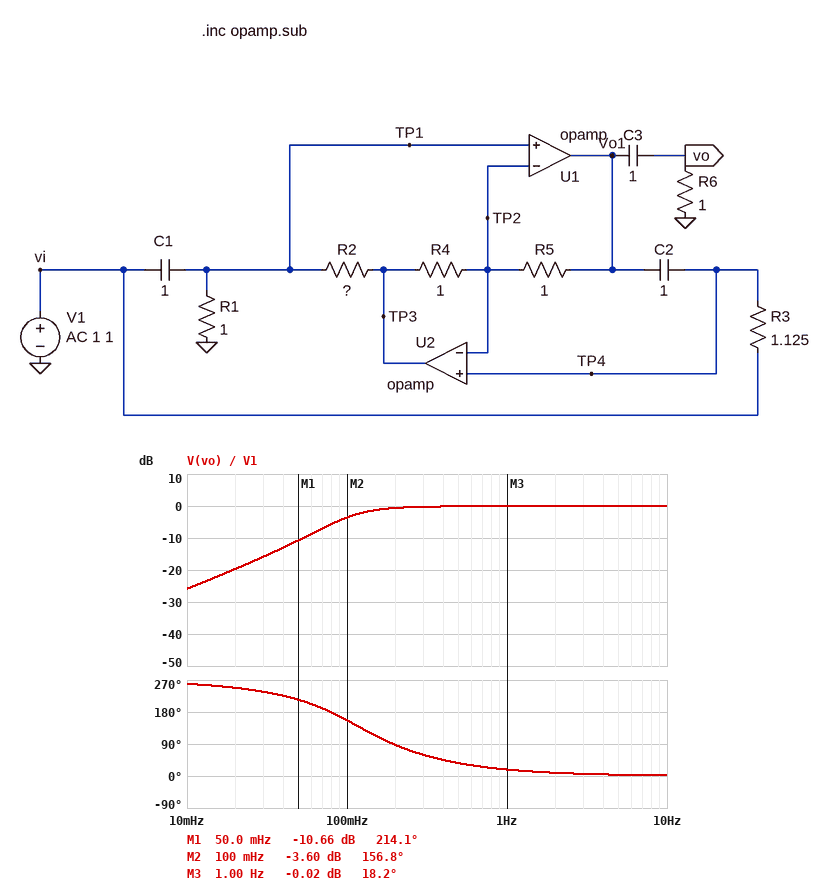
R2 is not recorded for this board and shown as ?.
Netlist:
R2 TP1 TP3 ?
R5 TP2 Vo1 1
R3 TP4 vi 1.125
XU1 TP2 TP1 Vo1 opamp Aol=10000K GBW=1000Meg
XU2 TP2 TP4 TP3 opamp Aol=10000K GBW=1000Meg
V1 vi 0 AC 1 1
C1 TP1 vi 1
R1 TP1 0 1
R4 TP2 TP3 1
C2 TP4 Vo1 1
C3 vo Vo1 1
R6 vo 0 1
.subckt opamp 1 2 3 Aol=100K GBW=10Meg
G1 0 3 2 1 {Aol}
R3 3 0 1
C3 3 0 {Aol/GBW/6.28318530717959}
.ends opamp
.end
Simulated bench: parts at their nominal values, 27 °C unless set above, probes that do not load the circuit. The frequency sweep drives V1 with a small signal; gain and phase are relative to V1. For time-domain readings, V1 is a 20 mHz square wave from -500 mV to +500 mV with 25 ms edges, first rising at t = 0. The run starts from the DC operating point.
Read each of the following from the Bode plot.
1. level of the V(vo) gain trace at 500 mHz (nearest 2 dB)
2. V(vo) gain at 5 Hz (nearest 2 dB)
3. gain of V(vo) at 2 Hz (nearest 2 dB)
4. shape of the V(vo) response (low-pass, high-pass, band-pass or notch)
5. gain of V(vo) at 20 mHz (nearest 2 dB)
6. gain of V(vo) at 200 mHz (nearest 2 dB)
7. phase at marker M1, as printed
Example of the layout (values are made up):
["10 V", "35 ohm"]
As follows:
["0 dB", "0 dB", "0 dB", "high-pass", "-20 dB", "0 dB", "214.1 deg"]
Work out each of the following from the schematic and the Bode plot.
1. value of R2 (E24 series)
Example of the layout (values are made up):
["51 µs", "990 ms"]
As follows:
["1.8 Ω"]
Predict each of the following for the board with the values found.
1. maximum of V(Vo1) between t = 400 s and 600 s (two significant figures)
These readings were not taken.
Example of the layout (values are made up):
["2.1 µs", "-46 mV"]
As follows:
["1.4 V"]
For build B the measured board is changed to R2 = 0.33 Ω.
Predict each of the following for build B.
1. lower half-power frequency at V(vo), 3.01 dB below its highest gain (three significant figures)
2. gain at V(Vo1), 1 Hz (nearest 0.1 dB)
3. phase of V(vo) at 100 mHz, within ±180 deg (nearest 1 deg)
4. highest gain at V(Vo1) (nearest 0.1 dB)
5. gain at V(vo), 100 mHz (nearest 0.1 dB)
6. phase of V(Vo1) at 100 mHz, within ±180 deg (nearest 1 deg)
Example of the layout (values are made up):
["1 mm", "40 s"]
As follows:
["293 mHz", "0.1 dB", "43 deg", "0.3 dB", "-10.0 dB", "-15 deg"]
